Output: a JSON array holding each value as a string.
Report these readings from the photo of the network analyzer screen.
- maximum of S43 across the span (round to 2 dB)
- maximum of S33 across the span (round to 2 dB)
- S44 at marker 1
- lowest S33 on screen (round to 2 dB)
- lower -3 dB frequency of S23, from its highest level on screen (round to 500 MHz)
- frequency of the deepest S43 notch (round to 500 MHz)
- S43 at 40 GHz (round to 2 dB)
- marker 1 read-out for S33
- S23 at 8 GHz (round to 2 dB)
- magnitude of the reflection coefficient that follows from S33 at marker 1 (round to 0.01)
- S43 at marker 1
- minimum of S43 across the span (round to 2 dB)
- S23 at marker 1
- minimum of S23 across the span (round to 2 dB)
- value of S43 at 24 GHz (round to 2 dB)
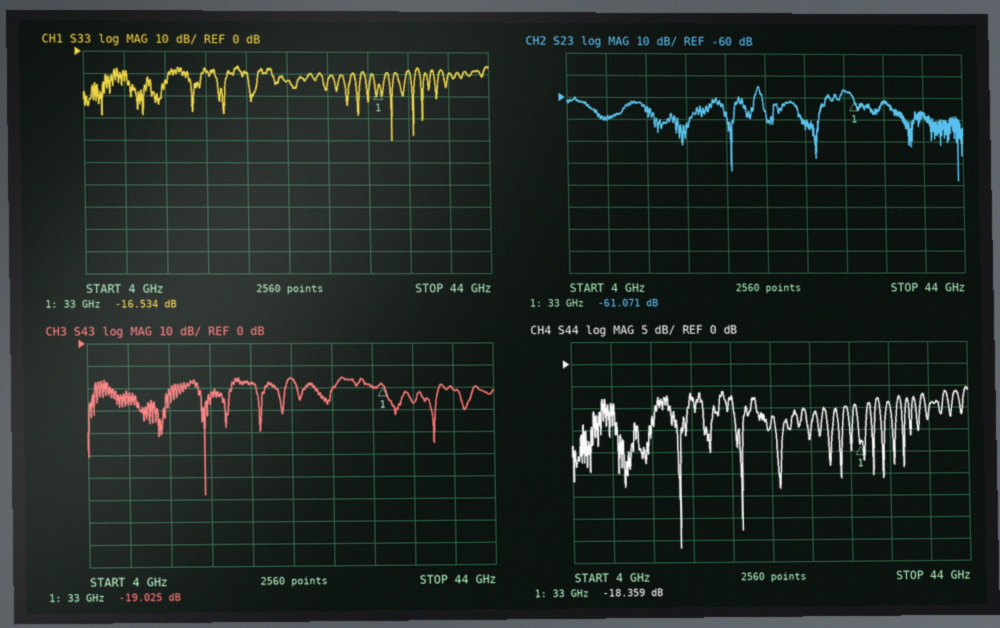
["-16 dB", "-6 dB", "-18.359 dB", "-40 dB", "23.0 GHz", "15.5 GHz", "-22 dB", "-16.534 dB", "-70 dB", "0.15", "-19.025 dB", "-68 dB", "-61.071 dB", "-98 dB", "-16 dB"]
